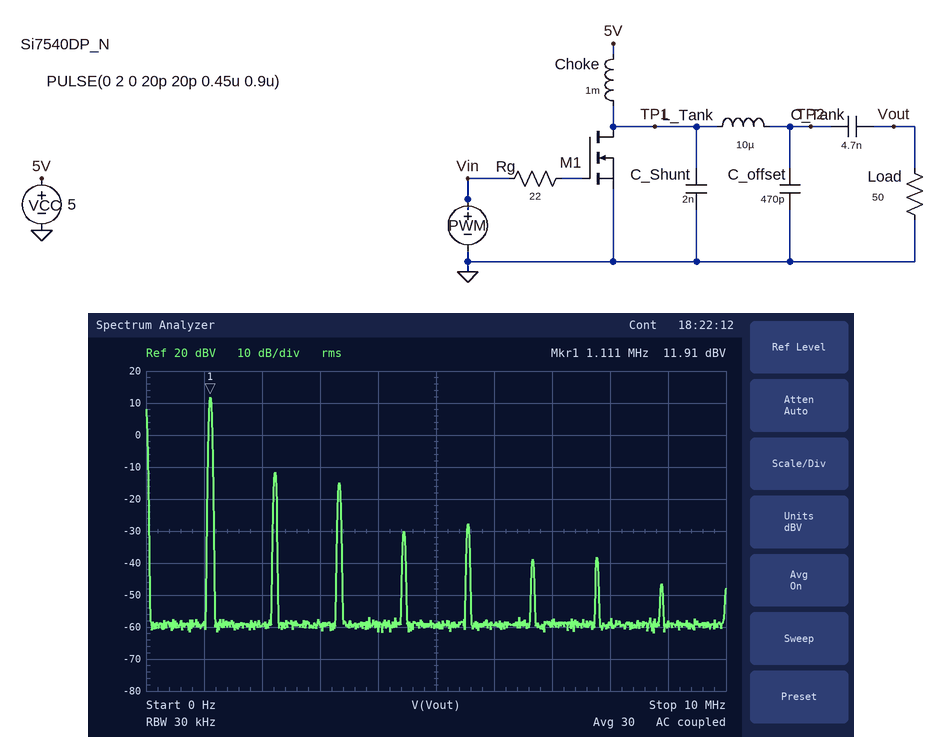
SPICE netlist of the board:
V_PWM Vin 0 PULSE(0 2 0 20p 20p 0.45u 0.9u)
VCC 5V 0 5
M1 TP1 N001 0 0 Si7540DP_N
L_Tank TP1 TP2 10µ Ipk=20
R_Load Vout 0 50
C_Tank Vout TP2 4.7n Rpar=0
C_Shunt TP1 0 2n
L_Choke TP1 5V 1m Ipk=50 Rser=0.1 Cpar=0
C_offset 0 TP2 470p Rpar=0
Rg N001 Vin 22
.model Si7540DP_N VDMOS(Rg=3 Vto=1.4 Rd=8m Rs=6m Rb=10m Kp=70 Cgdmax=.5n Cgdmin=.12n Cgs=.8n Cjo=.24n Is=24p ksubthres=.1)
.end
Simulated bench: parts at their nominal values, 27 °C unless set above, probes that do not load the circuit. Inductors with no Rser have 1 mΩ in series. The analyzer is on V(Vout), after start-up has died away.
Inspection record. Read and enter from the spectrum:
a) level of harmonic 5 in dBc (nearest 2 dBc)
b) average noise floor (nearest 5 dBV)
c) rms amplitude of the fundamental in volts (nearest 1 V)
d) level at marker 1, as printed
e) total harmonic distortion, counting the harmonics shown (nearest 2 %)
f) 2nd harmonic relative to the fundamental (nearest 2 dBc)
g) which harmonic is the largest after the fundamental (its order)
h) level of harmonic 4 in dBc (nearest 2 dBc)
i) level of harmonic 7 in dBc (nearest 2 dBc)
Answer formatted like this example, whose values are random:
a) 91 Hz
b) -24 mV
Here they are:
a) -40 dBc
b) -60 dBV
c) 4 V
d) 11.91 dBV
e) 8 %
f) -24 dBc
g) 2
h) -42 dBc
i) -50 dBc
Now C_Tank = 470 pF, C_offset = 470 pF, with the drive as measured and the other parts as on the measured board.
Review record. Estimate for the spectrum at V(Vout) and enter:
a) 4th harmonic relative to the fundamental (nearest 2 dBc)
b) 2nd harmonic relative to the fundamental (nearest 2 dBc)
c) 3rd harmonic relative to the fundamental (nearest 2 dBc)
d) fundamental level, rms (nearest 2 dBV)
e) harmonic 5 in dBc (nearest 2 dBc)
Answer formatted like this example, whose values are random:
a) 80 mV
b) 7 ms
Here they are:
a) -28 dBc
b) -4 dBc
c) -16 dBc
d) 4 dBV
e) -34 dBc
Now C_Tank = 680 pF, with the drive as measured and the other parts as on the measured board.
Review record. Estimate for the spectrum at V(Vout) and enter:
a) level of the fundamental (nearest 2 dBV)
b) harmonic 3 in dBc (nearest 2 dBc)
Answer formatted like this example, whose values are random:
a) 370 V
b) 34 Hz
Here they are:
a) 8 dBV
b) -20 dBc
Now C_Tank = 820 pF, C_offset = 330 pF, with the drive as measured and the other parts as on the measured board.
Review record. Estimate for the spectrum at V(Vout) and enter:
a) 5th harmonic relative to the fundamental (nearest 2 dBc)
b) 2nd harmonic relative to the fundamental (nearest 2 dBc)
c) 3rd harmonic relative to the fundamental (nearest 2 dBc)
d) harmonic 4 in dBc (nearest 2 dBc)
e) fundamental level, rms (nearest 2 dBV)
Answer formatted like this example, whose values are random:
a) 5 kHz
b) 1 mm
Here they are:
a) -36 dBc
b) -10 dBc
c) -20 dBc
d) -30 dBc
e) 8 dBV
